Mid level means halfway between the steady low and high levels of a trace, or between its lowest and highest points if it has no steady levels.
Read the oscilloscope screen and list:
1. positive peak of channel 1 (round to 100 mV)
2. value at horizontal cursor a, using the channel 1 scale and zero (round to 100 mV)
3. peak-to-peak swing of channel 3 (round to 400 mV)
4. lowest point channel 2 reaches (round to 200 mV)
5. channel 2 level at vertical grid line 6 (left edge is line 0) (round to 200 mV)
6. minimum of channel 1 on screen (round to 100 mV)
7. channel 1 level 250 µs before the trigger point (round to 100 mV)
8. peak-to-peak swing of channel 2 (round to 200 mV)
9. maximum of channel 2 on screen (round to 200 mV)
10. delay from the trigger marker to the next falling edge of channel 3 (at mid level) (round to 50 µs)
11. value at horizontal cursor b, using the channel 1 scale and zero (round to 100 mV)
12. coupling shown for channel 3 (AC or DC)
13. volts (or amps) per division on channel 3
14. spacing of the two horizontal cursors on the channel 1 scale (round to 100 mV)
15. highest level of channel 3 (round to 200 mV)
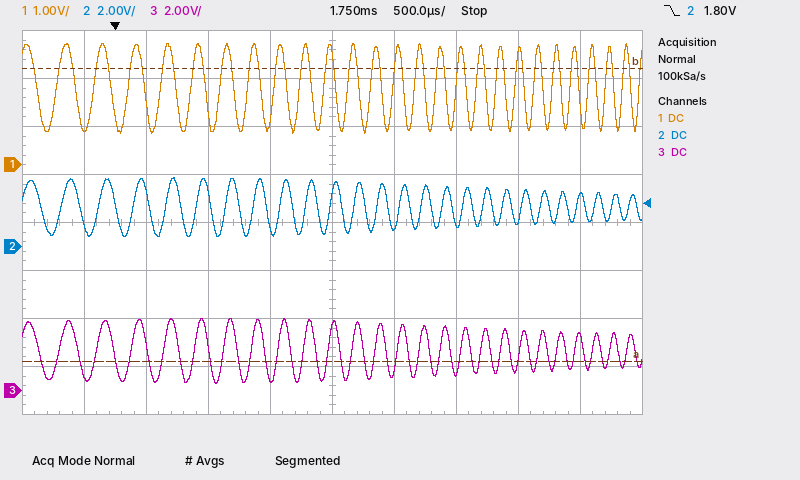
2.5 V
-4.1 V
2.8 V
400 mV
800 mV
700 mV
800 mV
2.4 V
2.8 V
250 µs
2.0 V
DC
2 V
6.1 V
3.0 V
